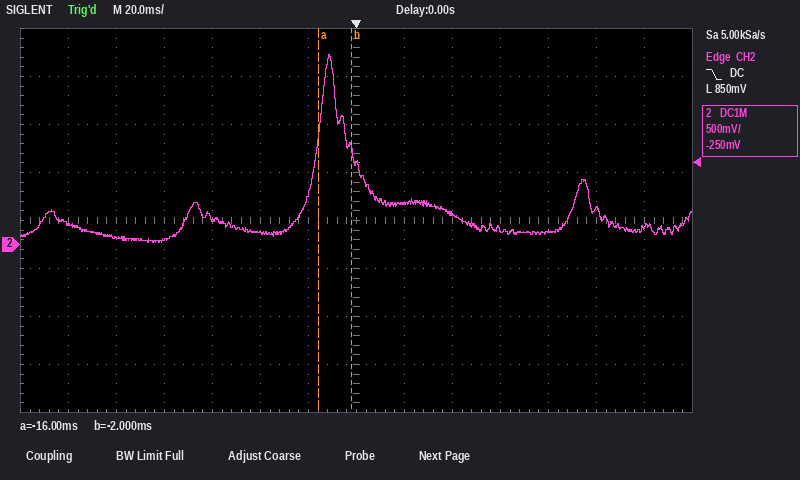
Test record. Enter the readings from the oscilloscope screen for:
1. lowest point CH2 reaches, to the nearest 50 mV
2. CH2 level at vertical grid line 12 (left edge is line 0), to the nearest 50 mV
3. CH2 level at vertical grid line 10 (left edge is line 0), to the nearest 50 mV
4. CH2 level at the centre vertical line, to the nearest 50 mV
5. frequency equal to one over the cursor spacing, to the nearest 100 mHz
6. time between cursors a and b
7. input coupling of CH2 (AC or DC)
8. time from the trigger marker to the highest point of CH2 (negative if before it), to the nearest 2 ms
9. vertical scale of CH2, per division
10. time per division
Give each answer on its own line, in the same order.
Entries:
0 mV
350 mV
150 mV
850 mV
71.4 Hz
14 ms
DC
-12 ms
500 mV
20 ms
